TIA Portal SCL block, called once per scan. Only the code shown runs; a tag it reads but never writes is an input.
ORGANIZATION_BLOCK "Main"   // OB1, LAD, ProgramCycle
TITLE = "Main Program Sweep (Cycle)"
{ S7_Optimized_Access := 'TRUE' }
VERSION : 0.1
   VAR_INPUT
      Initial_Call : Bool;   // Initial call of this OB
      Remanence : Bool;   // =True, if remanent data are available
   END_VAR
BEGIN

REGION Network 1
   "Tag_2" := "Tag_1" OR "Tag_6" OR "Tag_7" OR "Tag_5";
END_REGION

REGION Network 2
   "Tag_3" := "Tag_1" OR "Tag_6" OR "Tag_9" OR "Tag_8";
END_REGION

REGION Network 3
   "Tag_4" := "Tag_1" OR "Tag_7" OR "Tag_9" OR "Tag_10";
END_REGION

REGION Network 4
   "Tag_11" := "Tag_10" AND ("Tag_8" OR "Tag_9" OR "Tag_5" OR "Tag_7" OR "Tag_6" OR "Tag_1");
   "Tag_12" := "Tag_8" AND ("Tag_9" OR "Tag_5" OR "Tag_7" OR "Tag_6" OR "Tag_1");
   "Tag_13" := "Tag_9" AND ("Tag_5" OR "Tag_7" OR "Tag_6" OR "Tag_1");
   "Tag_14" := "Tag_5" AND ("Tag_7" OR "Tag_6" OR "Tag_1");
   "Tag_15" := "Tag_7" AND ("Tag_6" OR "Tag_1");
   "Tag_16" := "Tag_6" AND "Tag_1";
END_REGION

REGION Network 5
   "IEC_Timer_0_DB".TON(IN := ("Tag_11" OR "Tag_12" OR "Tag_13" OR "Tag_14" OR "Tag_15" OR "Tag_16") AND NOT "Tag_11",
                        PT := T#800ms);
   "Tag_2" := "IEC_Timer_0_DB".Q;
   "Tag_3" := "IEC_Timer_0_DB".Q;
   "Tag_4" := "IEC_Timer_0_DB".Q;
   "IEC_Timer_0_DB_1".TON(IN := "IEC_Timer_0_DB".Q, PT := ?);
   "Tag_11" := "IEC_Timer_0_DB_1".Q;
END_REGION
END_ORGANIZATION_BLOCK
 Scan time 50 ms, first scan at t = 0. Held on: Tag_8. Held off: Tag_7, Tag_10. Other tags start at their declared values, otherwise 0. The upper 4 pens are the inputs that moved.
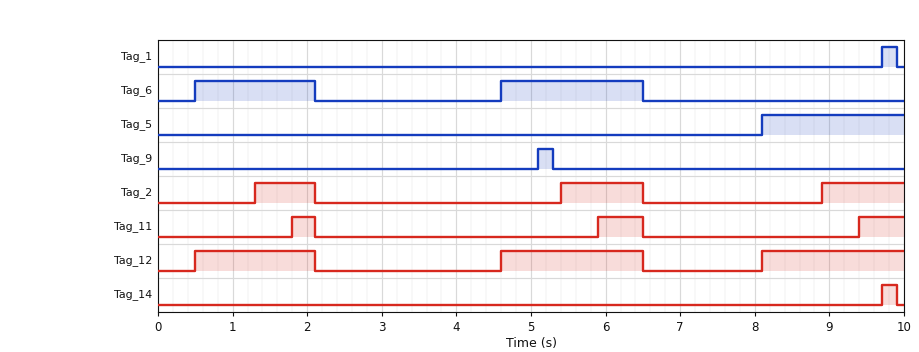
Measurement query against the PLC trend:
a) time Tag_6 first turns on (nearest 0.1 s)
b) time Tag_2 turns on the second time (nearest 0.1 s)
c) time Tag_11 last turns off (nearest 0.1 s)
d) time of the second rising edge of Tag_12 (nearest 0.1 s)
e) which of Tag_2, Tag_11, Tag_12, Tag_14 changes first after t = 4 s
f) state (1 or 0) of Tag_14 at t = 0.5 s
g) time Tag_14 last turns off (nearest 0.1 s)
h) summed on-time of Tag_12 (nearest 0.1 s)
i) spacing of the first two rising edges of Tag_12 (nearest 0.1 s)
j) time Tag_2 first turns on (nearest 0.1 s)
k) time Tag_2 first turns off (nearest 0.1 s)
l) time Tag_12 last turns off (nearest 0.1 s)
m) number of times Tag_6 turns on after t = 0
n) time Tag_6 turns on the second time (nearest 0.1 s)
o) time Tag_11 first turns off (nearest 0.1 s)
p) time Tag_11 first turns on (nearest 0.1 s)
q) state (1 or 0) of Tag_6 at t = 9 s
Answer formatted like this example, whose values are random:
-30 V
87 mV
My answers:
0.5 s
5.4 s
6.5 s
4.6 s
Tag_12
0
9.9 s
5.4 s
4.1 s
1.3 s
2.1 s
6.5 s
2
4.6 s
2.1 s
1.8 s
0
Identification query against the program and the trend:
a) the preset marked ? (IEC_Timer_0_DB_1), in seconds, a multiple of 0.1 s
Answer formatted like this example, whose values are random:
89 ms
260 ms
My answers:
0.5 s
